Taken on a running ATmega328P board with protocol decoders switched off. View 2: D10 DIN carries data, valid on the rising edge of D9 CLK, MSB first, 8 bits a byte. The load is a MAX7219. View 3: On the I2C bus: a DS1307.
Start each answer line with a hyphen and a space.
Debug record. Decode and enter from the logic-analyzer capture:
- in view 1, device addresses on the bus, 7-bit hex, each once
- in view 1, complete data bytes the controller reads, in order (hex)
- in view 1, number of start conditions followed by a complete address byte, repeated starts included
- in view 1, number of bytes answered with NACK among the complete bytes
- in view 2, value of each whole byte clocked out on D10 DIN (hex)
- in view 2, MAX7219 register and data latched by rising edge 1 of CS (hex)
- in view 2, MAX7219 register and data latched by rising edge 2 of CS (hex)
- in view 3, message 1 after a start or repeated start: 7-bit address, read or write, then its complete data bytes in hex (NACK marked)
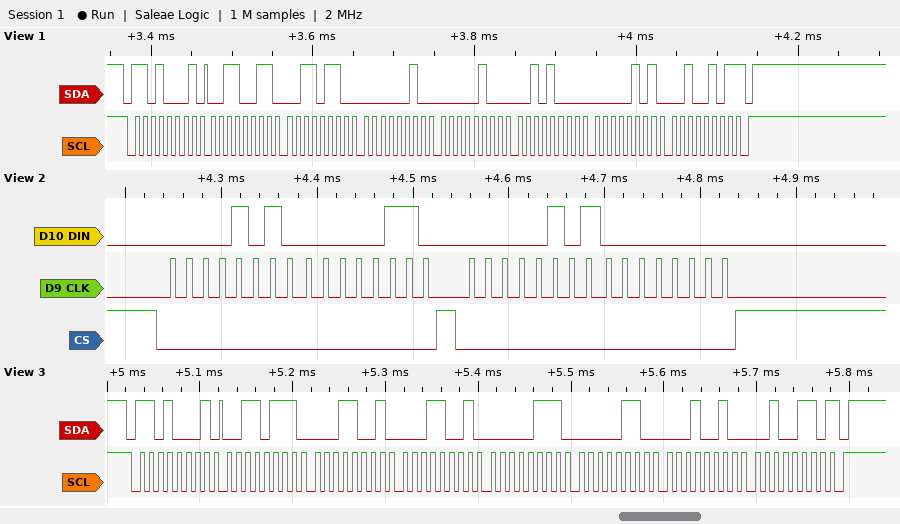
- 0x68
- 33 36 02 04 28 05 25
- 1
- 1
- 0A 06 05 00
- register 0xA, data 0x06
- register 0x5, data 0x00
- 0x68 read: 37 19 19 07 06 12 26 NACK
